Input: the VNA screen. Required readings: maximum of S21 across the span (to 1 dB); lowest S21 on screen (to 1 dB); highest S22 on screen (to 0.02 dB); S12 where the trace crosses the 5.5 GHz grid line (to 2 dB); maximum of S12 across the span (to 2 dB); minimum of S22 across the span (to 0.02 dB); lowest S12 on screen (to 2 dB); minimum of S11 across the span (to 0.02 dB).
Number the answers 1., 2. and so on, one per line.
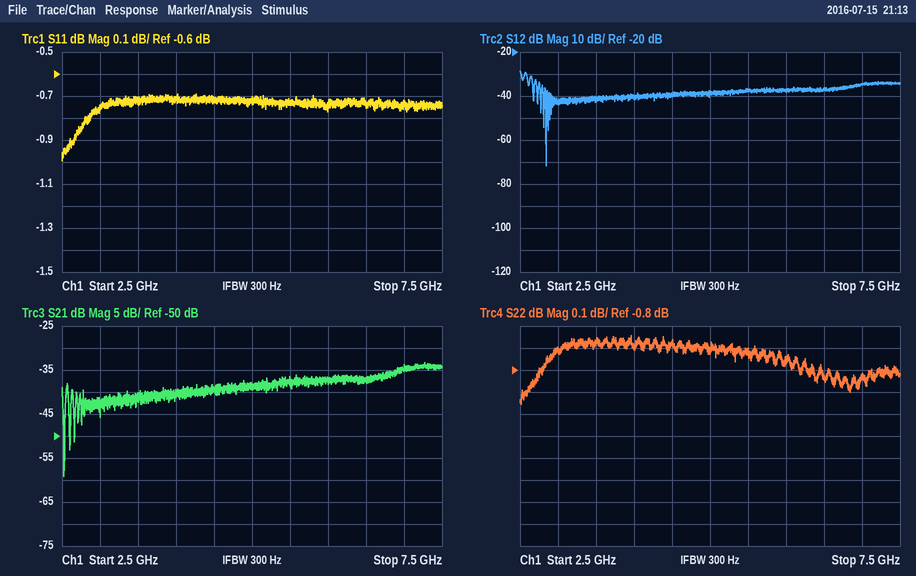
1. -33 dB
2. -59 dB
3. -0.64 dB
4. -38 dB
5. -28 dB
6. -0.96 dB
7. -72 dB
8. -1.00 dB
